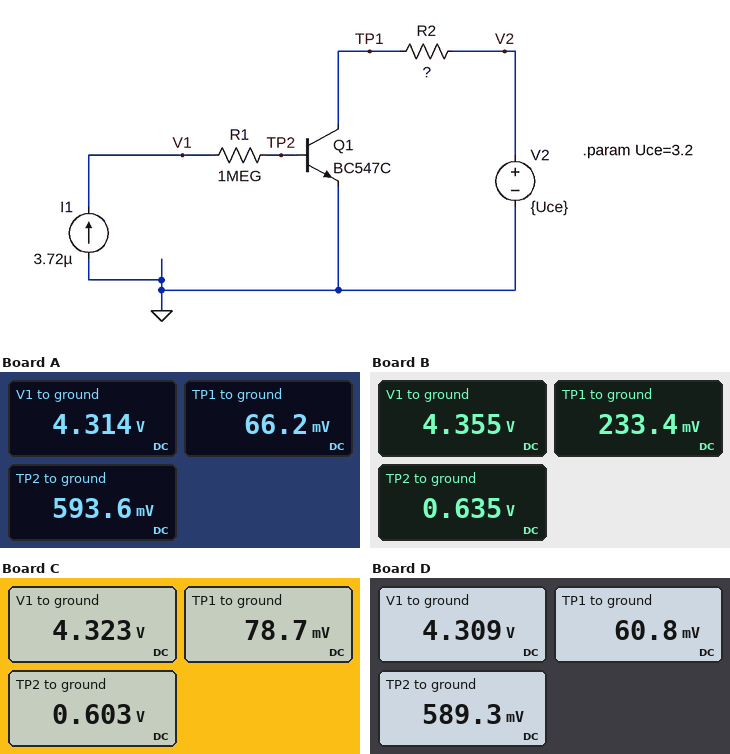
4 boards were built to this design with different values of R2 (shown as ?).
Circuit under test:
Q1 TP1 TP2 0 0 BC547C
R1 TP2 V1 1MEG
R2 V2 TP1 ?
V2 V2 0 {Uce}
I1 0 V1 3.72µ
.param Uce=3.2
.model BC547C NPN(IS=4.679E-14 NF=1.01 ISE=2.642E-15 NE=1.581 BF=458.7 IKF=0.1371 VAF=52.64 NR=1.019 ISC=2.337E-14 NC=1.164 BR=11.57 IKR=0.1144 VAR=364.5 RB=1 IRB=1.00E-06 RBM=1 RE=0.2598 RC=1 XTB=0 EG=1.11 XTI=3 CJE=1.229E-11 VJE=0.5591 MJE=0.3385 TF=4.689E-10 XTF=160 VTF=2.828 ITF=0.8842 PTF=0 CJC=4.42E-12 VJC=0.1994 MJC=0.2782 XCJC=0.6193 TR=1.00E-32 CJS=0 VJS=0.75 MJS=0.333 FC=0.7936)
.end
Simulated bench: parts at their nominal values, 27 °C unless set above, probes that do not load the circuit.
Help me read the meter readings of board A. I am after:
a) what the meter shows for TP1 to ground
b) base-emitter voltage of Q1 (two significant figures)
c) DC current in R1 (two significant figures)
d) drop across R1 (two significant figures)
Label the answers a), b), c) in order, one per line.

a) 66.2 mV
b) 590 mV
c) 3.7 µA
d) 3.7 V
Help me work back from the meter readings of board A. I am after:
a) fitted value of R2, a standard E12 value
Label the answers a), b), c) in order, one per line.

a) 10 kΩ
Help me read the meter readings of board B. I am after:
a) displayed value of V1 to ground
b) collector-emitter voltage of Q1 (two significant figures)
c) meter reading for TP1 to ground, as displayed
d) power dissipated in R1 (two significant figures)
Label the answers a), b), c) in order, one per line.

a) 4.355 V
b) 230 mV
c) 233.4 mV
d) 14 µW
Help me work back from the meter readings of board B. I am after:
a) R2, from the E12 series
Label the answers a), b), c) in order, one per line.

a) 1.8 kΩ
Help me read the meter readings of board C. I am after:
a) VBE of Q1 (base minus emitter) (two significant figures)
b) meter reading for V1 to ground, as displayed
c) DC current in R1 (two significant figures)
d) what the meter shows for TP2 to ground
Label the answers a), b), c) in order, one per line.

a) 600 mV
b) 4.323 V
c) 3.7 µA
d) 0.603 V
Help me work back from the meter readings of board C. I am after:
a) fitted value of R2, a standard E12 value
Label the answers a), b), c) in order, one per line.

a) 6.8 kΩ
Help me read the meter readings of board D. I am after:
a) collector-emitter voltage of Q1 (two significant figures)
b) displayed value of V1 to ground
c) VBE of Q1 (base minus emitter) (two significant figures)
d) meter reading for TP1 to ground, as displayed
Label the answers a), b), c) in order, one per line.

a) 61 mV
b) 4.309 V
c) 590 mV
d) 60.8 mV
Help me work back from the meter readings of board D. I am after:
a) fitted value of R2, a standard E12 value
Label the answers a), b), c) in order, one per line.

a) 12 kΩ
